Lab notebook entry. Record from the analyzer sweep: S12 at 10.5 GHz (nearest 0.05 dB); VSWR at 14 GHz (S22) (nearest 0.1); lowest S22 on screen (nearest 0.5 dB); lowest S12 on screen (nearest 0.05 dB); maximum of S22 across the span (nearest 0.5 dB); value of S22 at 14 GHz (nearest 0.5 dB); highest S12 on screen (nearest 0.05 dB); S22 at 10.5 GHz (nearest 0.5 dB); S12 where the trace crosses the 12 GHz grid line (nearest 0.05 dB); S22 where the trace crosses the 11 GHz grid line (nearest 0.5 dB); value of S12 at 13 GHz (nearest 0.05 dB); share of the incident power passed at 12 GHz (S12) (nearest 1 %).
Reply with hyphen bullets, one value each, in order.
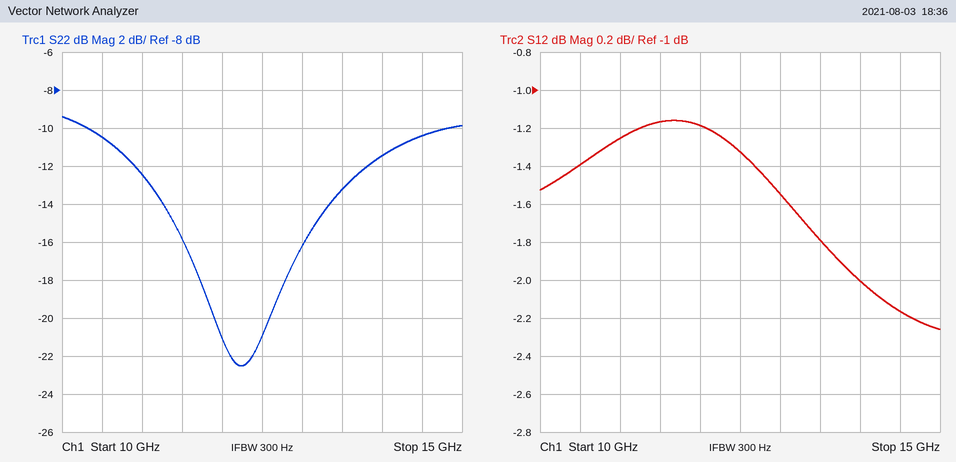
- -1.40 dB
- 1.7
- -22.5 dB
- -2.25 dB
- -9.5 dB
- -11.5 dB
- -1.15 dB
- -10.5 dB
- -1.20 dB
- -12.5 dB
- -1.55 dB
- 76 %
